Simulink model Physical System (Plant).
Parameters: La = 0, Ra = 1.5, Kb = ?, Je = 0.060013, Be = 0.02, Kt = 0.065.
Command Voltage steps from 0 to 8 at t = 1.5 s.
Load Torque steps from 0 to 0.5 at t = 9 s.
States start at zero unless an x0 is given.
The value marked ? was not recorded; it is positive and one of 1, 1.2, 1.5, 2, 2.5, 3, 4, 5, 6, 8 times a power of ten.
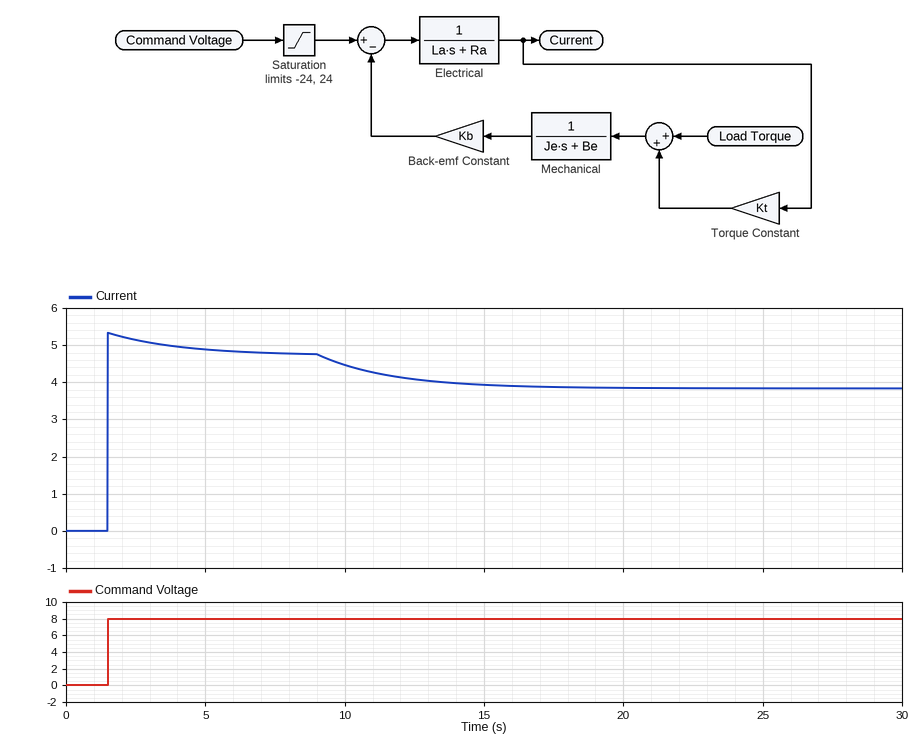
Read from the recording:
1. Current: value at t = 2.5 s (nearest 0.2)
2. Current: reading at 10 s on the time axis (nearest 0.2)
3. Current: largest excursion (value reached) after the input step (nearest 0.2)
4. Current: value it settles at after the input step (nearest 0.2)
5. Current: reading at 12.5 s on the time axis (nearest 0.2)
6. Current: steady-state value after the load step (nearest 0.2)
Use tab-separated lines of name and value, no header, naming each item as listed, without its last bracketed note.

Current: value at t = 2.5 s	5.2
Current: reading at 10 s on the time axis	4.4
Current: largest excursion (value reached) after the input step	5.4
Current: value it settles at after the input step	4.8
Current: reading at 12.5 s on the time axis	4.0
Current: steady-state value after the load step	3.8
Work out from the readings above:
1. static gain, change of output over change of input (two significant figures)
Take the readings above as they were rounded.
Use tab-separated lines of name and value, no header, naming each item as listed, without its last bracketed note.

static gain, change of output over change of input	0.60
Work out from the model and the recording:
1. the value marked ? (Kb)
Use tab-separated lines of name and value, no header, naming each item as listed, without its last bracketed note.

the value marked ?	0.06
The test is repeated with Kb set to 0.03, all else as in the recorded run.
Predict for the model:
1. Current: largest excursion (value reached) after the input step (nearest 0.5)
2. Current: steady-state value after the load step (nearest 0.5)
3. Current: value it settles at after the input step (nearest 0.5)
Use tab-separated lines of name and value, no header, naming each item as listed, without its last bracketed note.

Current: largest excursion (value reached) after the input step	5.5
Current: steady-state value after the load step	4.5
Current: value it settles at after the input step	5.0
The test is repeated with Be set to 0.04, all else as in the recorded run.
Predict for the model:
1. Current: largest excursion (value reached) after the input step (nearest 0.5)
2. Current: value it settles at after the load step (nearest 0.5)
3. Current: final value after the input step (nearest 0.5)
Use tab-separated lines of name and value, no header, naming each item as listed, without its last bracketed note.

Current: largest excursion (value reached) after the input step	5.5
Current: value it settles at after the load step	4.5
Current: final value after the input step	5.0
